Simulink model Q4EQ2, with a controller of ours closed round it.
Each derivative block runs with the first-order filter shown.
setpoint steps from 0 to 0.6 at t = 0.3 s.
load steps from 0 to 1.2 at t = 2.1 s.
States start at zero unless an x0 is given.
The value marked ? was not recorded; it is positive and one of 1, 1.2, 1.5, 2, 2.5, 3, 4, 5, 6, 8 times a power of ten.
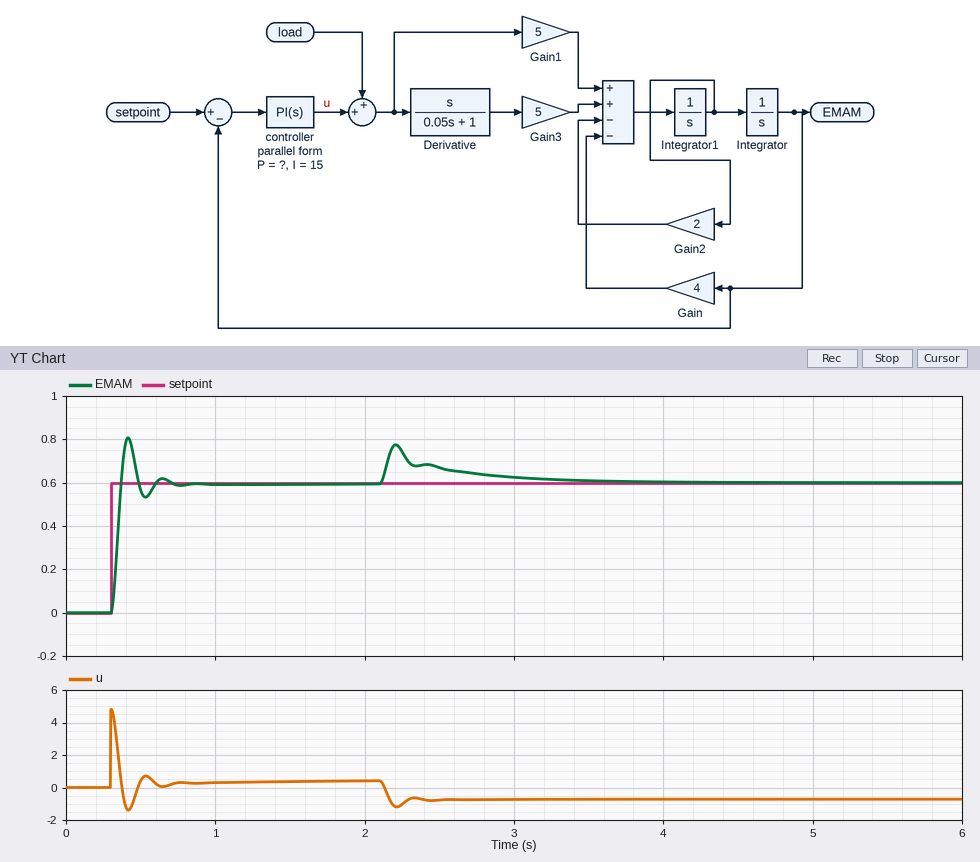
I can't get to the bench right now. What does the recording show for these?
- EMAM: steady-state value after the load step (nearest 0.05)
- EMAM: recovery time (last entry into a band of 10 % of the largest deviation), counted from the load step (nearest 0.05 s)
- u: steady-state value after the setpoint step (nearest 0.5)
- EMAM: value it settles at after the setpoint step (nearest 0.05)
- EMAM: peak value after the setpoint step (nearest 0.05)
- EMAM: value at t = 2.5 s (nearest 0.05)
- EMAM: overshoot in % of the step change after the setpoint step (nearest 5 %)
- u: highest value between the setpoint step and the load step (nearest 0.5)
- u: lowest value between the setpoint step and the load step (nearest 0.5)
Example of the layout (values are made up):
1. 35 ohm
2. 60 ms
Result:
1. 0.60
2. 1.05 s
3. 0.5
4. 0.60
5. 0.80
6. 0.65
7. 35 %
8. 5.0
9. -1.5
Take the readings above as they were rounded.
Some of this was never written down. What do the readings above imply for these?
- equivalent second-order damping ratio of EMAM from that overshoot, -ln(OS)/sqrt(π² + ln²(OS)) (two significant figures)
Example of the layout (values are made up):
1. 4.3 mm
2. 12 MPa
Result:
1. 0.32
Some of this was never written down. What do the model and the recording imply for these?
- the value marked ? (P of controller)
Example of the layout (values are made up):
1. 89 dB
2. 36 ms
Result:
1. 8
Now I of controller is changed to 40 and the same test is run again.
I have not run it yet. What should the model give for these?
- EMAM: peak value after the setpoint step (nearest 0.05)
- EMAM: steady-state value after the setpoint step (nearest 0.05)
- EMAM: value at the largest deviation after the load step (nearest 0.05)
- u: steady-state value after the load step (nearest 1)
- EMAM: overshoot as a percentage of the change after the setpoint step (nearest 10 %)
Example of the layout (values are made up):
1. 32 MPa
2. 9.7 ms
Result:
1. 0.90
2. 0.60
3. 0.75
4. -1
5. 50 %
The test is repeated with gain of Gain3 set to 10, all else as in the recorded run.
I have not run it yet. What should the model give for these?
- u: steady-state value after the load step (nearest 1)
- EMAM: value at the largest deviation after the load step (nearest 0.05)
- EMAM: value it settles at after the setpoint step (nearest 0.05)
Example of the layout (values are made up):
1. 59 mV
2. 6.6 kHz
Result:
1. -1
2. 0.80
3. 0.60
